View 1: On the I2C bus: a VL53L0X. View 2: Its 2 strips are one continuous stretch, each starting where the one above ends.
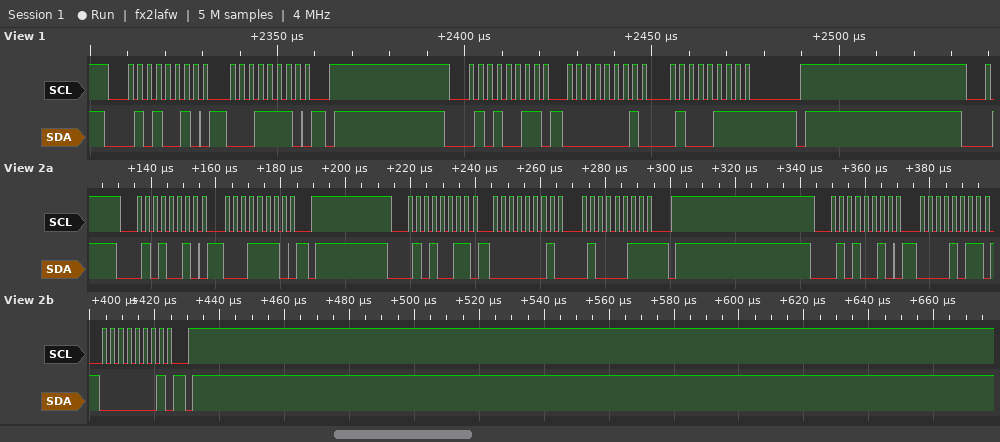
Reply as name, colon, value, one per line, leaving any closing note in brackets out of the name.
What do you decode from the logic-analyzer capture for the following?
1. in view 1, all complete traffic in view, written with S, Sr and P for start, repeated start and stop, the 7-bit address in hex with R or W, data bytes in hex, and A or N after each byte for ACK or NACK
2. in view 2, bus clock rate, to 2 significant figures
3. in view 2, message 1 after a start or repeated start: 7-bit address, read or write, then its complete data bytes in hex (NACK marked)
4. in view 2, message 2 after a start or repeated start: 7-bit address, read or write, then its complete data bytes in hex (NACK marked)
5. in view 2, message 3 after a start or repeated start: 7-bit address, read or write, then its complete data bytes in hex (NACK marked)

in view 1, all complete traffic in view, written with S, Sr and P for start, repeated start and stop, the 7-bit address in hex with R or W, data bytes in hex, and A or N after each byte for ACK or NACK: S 29W A 1E A P S 29R A 01 A 47 N P
in view 2, bus clock rate, to 2 significant figures: 400 kHz
in view 2, message 1 after a start or repeated start: 7-bit address, read or write, then its complete data bytes in hex: 0x29 write: 1E
in view 2, message 2 after a start or repeated start: 7-bit address, read or write, then its complete data bytes in hex: 0x29 read: 01 43 NACK
in view 2, message 3 after a start or repeated start: 7-bit address, read or write, then its complete data bytes in hex: 0x29 write: 0B 01
